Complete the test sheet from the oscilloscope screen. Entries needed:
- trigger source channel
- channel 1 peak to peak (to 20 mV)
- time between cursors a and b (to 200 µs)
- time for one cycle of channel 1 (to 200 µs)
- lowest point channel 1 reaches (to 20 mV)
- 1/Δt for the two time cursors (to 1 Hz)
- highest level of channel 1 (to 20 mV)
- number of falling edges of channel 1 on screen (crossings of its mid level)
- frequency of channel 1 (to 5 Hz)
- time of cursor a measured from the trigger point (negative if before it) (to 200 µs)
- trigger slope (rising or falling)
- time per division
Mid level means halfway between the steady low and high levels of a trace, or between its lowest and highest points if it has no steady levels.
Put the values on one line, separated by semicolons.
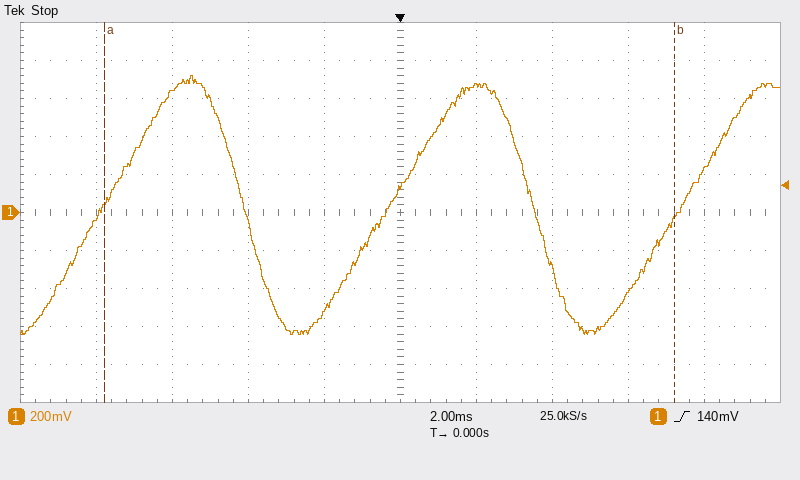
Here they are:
channel 1; 1.36 V; 15.0 ms; 7.6 ms; -640 mV; 67 Hz; 720 mV; 2; 130 Hz; -7.8 ms; rising; 2 ms
